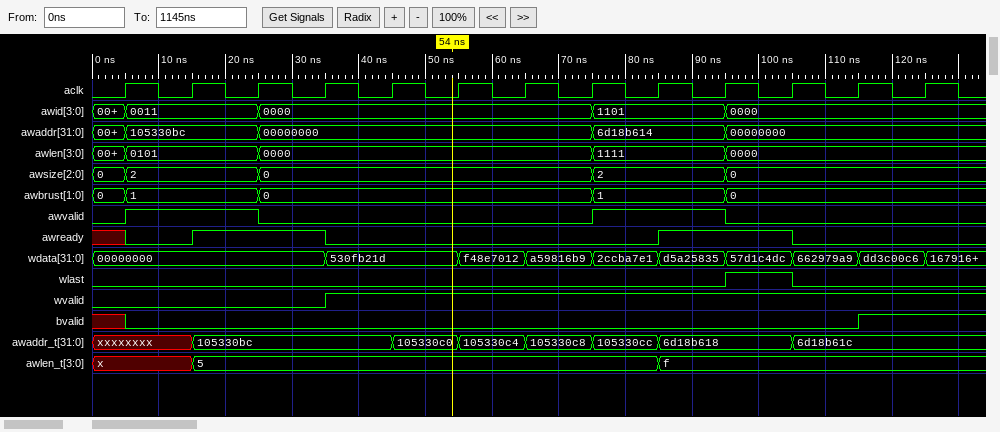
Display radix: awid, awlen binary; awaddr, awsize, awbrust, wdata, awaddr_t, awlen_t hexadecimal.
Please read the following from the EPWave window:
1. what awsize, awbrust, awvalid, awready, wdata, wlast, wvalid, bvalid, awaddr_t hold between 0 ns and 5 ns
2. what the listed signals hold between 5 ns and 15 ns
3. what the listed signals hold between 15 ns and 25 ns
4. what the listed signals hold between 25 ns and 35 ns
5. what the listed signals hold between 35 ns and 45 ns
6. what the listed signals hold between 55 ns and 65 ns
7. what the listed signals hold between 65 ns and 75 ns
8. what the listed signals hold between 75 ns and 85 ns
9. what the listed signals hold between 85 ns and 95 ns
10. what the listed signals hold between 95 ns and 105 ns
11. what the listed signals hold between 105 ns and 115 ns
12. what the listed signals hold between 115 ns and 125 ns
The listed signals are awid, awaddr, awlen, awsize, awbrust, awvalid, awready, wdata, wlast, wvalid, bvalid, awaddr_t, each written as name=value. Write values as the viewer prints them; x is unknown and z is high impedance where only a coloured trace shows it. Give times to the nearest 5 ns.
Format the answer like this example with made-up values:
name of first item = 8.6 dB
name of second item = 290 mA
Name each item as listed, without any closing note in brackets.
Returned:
what awsize, awbrust, awvalid, awready, wdata, wlast, wvalid, bvalid, awaddr_t hold between 0 ns and 5 ns = awsize=0, awbrust=0, awvalid=0, awready=x, wdata=00000000, wlast=0, wvalid=0, bvalid=x, awaddr_t=xxxxxxxx
what the listed signals hold between 5 ns and 15 ns = awid=0011, awaddr=105330bc, awlen=0101, awsize=2, awbrust=1, awvalid=1, awready=0, wdata=00000000, wlast=0, wvalid=0, bvalid=0, awaddr_t=xxxxxxxx
what the listed signals hold between 15 ns and 25 ns = awid=0011, awaddr=105330bc, awlen=0101, awsize=2, awbrust=1, awvalid=1, awready=1, wdata=00000000, wlast=0, wvalid=0, bvalid=0, awaddr_t=105330bc
what the listed signals hold between 25 ns and 35 ns = awid=0000, awaddr=00000000, awlen=0000, awsize=0, awbrust=0, awvalid=0, awready=1, wdata=00000000, wlast=0, wvalid=0, bvalid=0, awaddr_t=105330bc
what the listed signals hold between 35 ns and 45 ns = awid=0000, awaddr=00000000, awlen=0000, awsize=0, awbrust=0, awvalid=0, awready=0, wdata=530fb21d, wlast=0, wvalid=1, bvalid=0, awaddr_t=105330bc
what the listed signals hold between 55 ns and 65 ns = awid=0000, awaddr=00000000, awlen=0000, awsize=0, awbrust=0, awvalid=0, awready=0, wdata=f48e7012, wlast=0, wvalid=1, bvalid=0, awaddr_t=105330c4
what the listed signals hold between 65 ns and 75 ns = awid=0000, awaddr=00000000, awlen=0000, awsize=0, awbrust=0, awvalid=0, awready=0, wdata=a59816b9, wlast=0, wvalid=1, bvalid=0, awaddr_t=105330c8
what the listed signals hold between 75 ns and 85 ns = awid=1101, awaddr=6d18b614, awlen=1111, awsize=2, awbrust=1, awvalid=1, awready=0, wdata=2ccba7e1, wlast=0, wvalid=1, bvalid=0, awaddr_t=105330cc
what the listed signals hold between 85 ns and 95 ns = awid=1101, awaddr=6d18b614, awlen=1111, awsize=2, awbrust=1, awvalid=1, awready=1, wdata=d5a25835, wlast=0, wvalid=1, bvalid=0, awaddr_t=6d18b618
what the listed signals hold between 95 ns and 105 ns = awid=0000, awaddr=00000000, awlen=0000, awsize=0, awbrust=0, awvalid=0, awready=1, wdata=57d1c4dc, wlast=1, wvalid=1, bvalid=0, awaddr_t=6d18b618
what the listed signals hold between 105 ns and 115 ns = awid=0000, awaddr=00000000, awlen=0000, awsize=0, awbrust=0, awvalid=0, awready=0, wdata=662979a9, wlast=0, wvalid=1, bvalid=0, awaddr_t=6d18b61c
what the listed signals hold between 115 ns and 125 ns = awid=0000, awaddr=00000000, awlen=0000, awsize=0, awbrust=0, awvalid=0, awready=0, wdata=dd3c00c6, wlast=0, wvalid=1, bvalid=1, awaddr_t=6d18b61c
